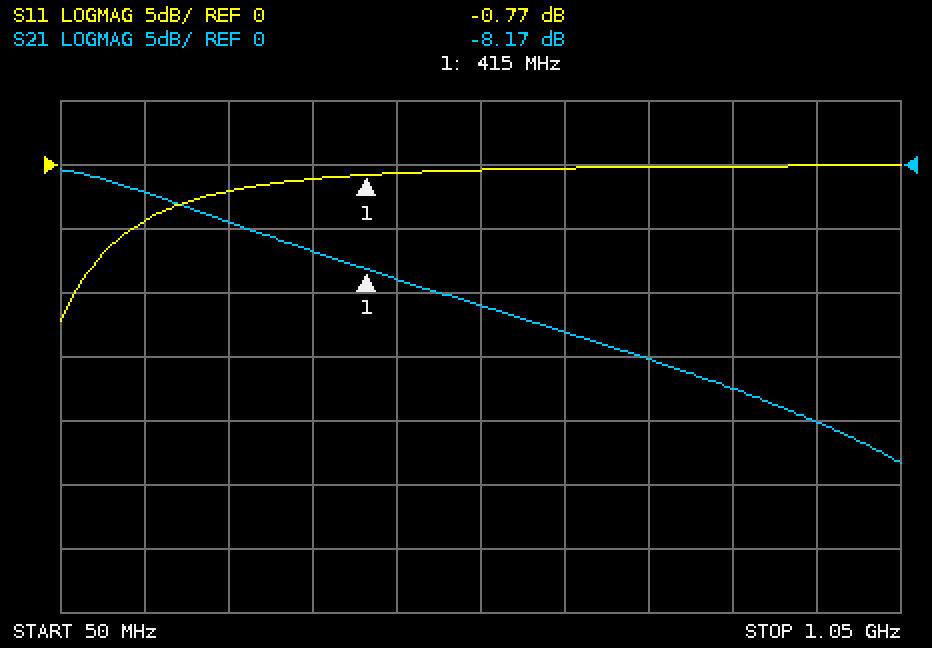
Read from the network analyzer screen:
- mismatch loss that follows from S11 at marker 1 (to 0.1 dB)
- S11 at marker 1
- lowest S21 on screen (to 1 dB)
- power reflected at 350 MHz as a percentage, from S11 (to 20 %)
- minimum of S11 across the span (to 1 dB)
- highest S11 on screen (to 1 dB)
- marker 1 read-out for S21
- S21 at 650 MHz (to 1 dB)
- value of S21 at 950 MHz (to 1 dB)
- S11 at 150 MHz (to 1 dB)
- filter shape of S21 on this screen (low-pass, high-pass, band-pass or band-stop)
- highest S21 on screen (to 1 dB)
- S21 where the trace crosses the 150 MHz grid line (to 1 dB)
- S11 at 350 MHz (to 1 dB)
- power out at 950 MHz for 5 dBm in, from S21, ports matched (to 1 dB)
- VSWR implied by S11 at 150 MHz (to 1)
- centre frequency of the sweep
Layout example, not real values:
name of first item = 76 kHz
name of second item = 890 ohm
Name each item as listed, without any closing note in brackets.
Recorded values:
mismatch loss that follows from S11 at marker 1 = 7.9 dB
S11 at marker 1 = -0.77 dB
lowest S21 on screen = -23 dB
power reflected at 350 MHz as a percentage, from S11 = 80 %
minimum of S11 across the span = -12 dB
highest S11 on screen = 0 dB
marker 1 read-out for S21 = -8.17 dB
S21 at 650 MHz = -13 dB
value of S21 at 950 MHz = -20 dB
S11 at 150 MHz = -4 dB
filter shape of S21 on this screen = low-pass
highest S21 on screen = 0 dB
S21 where the trace crosses the 150 MHz grid line = -2 dB
S11 at 350 MHz = -1 dB
power out at 950 MHz for 5 dBm in, from S21, ports matched = -15 dBm
VSWR implied by S11 at 150 MHz = 4
centre frequency of the sweep = 550 MHz
